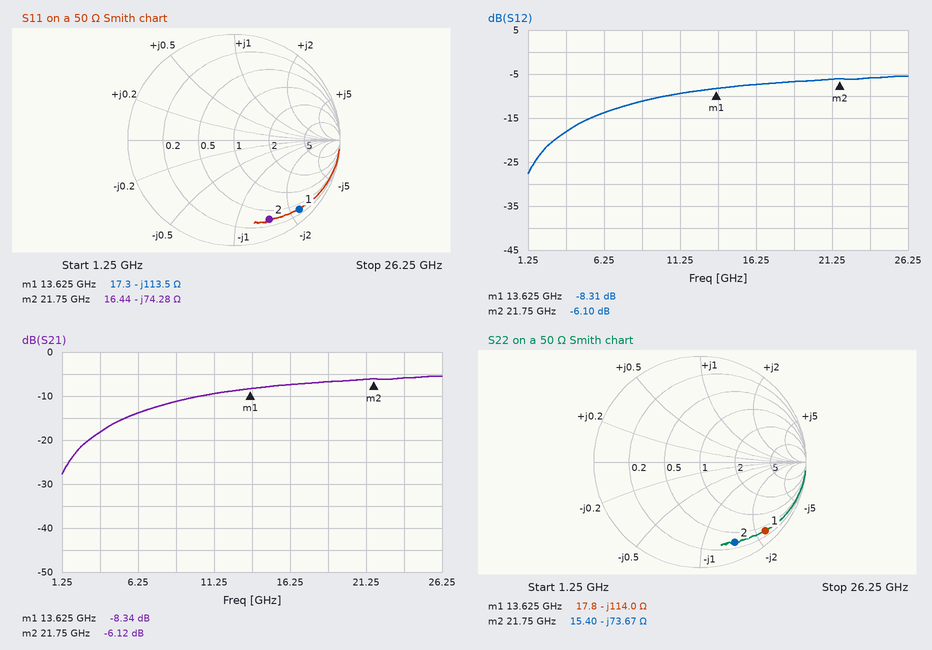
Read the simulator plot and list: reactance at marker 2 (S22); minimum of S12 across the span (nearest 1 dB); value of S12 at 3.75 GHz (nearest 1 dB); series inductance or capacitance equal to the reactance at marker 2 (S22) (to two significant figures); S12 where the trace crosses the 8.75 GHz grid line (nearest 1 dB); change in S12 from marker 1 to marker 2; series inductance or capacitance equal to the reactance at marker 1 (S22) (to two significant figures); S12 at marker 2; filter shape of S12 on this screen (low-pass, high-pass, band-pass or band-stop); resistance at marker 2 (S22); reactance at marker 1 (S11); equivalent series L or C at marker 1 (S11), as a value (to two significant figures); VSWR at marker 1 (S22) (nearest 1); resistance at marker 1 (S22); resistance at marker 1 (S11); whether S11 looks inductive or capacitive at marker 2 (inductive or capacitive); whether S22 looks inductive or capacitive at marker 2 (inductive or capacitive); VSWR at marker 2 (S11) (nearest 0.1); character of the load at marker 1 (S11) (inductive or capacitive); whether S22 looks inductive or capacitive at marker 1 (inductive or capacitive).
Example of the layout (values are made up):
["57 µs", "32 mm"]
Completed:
["-73.67 Ω", "-28 dB", "-18 dB", "99 fF", "-11 dB", "2.21 dB", "100 fF", "-6.10 dB", "high-pass", "15.40 Ω", "-113.5 Ω", "100 fF", "18", "17.8 Ω", "17.3 Ω", "capacitive", "capacitive", "10.0", "capacitive", "capacitive"]
